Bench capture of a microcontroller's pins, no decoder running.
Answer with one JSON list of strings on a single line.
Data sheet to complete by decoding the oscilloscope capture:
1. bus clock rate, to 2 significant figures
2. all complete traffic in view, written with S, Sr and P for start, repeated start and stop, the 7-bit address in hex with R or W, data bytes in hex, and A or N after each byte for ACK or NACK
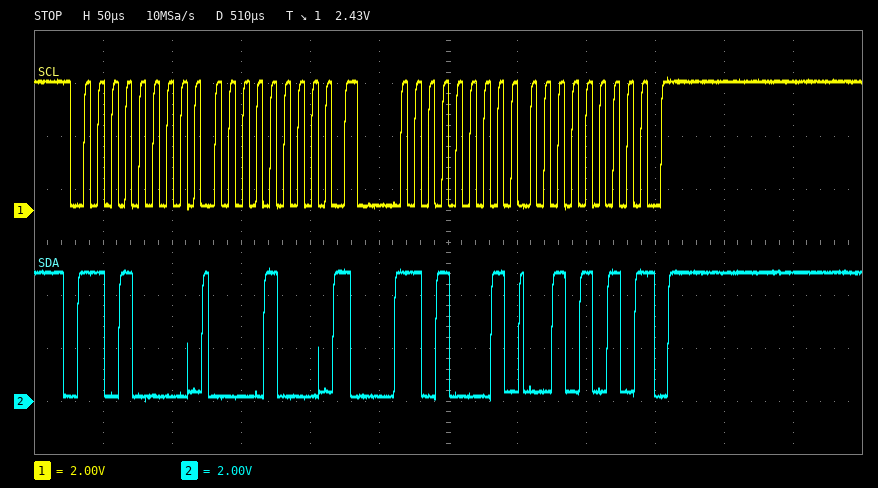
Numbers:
["100 kHz", "S 68W A 08 A Sr 68R A 2A N P"]
